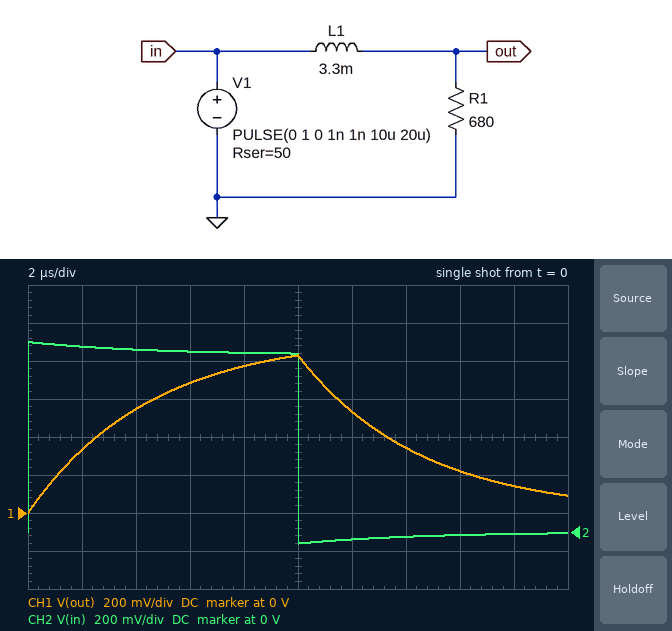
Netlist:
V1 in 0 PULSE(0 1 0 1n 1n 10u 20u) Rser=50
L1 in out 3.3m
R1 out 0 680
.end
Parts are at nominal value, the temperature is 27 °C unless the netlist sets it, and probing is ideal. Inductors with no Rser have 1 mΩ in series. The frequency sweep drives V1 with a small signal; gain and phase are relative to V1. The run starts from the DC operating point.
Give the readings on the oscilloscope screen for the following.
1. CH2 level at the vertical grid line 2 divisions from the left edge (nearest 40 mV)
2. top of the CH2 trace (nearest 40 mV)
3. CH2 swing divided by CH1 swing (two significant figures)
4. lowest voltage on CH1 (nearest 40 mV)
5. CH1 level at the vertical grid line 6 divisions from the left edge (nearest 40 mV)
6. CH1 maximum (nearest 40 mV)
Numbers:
960 mV
1.00 V
1.3
0 V
520 mV
840 mV
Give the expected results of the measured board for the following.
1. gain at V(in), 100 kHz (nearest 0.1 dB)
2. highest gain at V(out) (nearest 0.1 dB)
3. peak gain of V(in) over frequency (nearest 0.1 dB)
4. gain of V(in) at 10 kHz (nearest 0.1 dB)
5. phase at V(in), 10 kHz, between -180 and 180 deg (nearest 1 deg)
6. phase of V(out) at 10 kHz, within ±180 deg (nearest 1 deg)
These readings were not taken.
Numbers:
-0.1 dB
-0.6 dB
0 dB
-0.6 dB
1 deg
-16 deg
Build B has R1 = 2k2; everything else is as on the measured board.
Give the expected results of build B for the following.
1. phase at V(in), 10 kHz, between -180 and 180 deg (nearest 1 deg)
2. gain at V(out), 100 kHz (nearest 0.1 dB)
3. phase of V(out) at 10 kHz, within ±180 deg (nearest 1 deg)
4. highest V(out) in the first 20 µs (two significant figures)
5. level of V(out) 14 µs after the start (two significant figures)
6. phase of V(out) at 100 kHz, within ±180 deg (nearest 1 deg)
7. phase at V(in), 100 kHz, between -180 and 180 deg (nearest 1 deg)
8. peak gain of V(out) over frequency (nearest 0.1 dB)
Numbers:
0 deg
-2.9 dB
-5 deg
980 mV
64 mV
-43 deg
1 deg
-0.2 dB
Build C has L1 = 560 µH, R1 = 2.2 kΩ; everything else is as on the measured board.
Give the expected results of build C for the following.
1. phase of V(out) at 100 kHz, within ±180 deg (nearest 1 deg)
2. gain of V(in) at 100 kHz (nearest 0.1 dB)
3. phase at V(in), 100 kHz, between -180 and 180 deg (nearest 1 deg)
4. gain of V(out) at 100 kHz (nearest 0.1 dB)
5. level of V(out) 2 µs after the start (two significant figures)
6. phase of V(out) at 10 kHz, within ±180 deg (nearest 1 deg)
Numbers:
-9 deg
-0.2 dB
0 deg
-0.3 dB
980 mV
-1 deg
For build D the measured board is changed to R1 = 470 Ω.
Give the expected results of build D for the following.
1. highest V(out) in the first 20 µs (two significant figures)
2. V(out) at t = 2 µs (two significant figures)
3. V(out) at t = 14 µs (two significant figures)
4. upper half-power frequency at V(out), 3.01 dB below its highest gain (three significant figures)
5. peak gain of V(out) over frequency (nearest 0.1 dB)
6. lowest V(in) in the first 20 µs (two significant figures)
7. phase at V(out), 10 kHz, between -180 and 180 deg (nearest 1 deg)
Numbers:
720 mV
240 mV
380 mV
25.1 kHz
-0.9 dB
-76 mV
-22 deg
